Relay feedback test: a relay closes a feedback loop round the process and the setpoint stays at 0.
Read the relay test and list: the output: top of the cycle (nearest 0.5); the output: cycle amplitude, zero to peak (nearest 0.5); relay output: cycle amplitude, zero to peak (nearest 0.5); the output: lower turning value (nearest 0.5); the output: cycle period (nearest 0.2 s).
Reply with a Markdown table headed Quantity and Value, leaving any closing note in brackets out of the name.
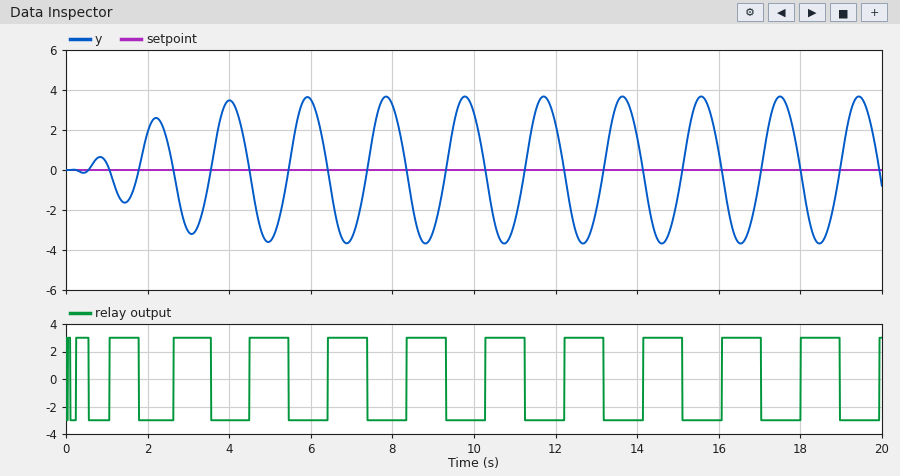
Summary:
| Quantity | Value |
|---|---|
| the output: top of the cycle | 3.5 |
| the output: cycle amplitude, zero to peak | 3.5 |
| relay output: cycle amplitude, zero to peak | 3.0 |
| the output: lower turning value | -3.5 |
| the output: cycle period | 2.0 s |
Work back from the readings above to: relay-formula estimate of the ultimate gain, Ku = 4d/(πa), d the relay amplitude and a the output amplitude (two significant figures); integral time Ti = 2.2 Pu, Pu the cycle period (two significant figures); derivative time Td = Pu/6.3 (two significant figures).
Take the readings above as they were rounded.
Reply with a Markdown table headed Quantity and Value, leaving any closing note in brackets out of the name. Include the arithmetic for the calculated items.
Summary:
| Quantity | Value |
|---|---|
| relay-formula estimate of the ultimate gain, Ku = 4d/(πa), d the relay amplitude and a the output amplitude | 4 × 3 / (π × 3.5) = 1.1 |
| integral time Ti = 2.2 Pu, Pu the cycle period | 2.2 × 2 = 4.4 s |
| derivative time Td = Pu/6.3 | 2 / 6.3 = 0.32 s |
